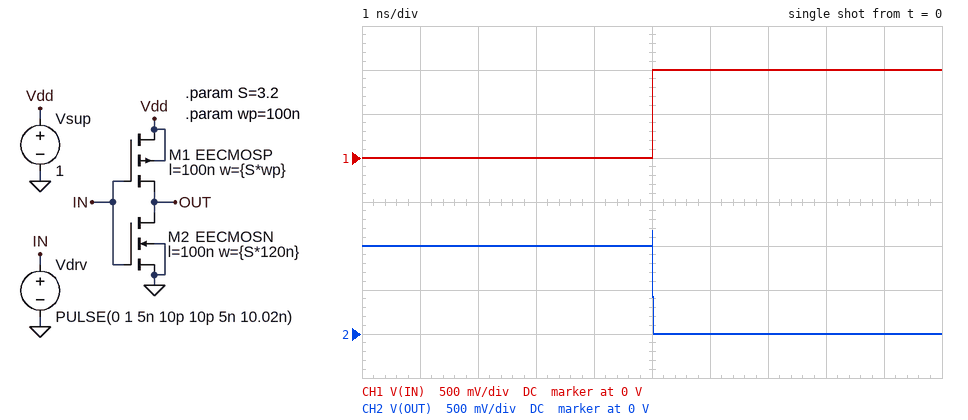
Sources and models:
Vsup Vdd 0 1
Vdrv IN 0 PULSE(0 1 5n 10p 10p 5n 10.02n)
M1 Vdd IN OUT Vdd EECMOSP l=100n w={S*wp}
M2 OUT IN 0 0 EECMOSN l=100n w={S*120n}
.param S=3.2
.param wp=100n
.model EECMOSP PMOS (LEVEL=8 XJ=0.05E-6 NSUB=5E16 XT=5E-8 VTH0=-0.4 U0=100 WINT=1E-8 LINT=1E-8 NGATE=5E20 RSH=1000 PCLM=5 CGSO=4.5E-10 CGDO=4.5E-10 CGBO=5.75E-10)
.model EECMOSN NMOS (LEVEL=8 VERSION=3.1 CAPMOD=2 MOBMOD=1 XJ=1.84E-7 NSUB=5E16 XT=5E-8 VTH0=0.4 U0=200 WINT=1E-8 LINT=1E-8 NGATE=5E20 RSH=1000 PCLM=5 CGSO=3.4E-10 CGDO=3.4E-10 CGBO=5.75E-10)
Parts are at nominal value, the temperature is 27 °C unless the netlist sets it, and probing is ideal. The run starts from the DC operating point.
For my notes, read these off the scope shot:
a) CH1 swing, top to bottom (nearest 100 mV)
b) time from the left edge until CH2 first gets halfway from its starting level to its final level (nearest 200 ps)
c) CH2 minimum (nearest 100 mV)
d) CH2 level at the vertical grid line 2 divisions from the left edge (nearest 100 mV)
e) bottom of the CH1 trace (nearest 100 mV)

1.0 V
5.0 ns
0 V
1.0 V
0 V
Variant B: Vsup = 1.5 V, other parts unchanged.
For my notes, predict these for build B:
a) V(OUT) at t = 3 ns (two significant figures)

1.5 V
